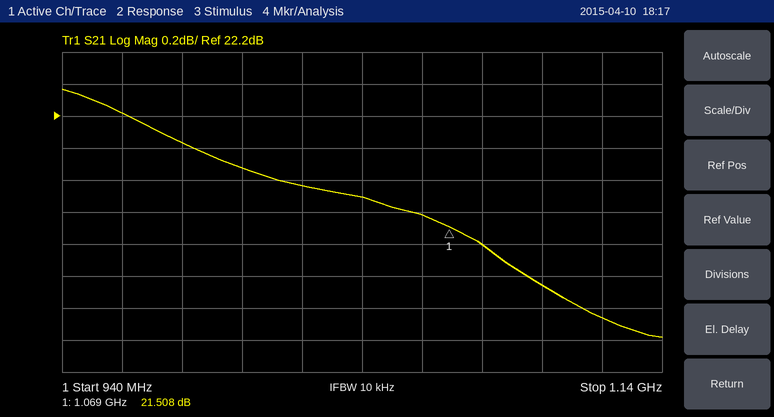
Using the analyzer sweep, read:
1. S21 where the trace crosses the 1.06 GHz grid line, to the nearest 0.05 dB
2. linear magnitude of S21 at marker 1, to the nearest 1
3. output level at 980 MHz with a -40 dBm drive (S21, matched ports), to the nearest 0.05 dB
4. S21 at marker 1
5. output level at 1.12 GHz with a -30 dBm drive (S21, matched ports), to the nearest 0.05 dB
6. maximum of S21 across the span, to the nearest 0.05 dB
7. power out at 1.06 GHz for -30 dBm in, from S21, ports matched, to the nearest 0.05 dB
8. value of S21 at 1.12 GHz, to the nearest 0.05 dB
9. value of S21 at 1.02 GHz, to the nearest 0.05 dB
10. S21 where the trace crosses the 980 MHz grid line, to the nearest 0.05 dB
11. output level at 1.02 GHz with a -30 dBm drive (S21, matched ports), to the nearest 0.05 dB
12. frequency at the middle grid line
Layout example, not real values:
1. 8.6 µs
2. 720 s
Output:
1. 21.60 dB
2. 12
3. -17.95 dBm
4. 21.508 dB
5. -9.05 dBm
6. 22.35 dB
7. -8.40 dBm
8. 20.95 dB
9. 21.75 dB
10. 22.05 dB
11. -8.25 dBm
12. 1.04 GHz
